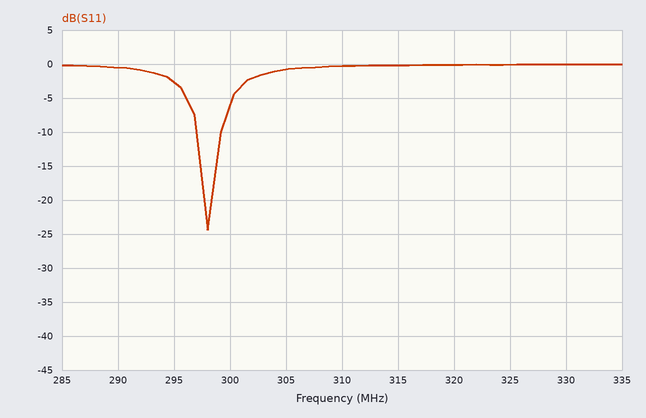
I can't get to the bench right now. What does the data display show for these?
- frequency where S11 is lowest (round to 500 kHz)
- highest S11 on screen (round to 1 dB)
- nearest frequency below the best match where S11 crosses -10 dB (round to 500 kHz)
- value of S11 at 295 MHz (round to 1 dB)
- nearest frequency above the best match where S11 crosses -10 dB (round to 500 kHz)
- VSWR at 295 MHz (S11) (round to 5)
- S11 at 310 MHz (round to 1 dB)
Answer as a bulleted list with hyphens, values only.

- 298.0 MHz
- 0 dB
- 297.0 MHz
- -3 dB
- 299.0 MHz
- 5
- 0 dB
